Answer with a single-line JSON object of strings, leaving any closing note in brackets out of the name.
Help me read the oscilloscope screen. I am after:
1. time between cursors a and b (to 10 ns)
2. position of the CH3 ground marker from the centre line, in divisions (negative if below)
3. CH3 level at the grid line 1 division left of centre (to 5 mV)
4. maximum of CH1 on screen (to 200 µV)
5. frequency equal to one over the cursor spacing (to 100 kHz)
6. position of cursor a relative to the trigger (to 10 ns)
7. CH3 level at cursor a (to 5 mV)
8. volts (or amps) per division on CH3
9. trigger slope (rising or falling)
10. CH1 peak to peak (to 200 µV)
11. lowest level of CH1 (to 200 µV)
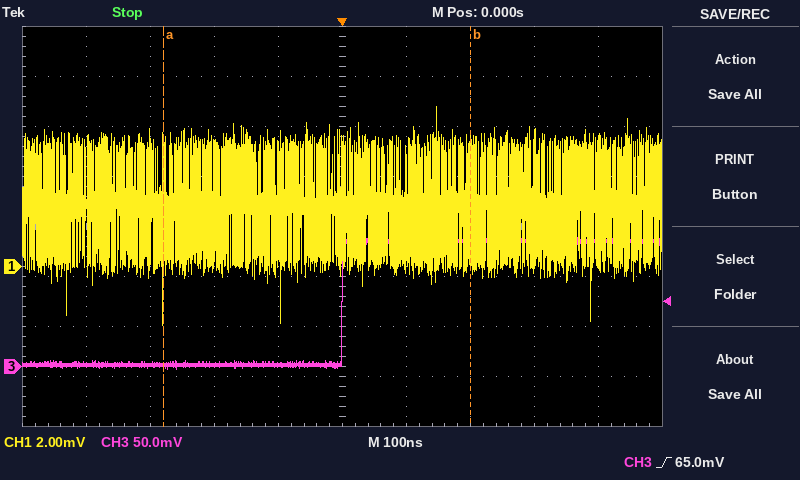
{"time between cursors a and b": "480 ns", "position of the CH3 ground marker from the centre line, in divisions": "-2.8 div", "CH3 level at the grid line 1 division left of centre": "0 mV", "maximum of CH1 on screen": "6.4 mV", "frequency equal to one over the cursor spacing": "2.1 MHz", "position of cursor a relative to the trigger": "-280 ns", "CH3 level at cursor a": "0 mV", "volts (or amps) per division on CH3": "50 mV", "trigger slope": "rising", "CH1 peak to peak": "8.8 mV", "lowest level of CH1": "-2.4 mV"}
